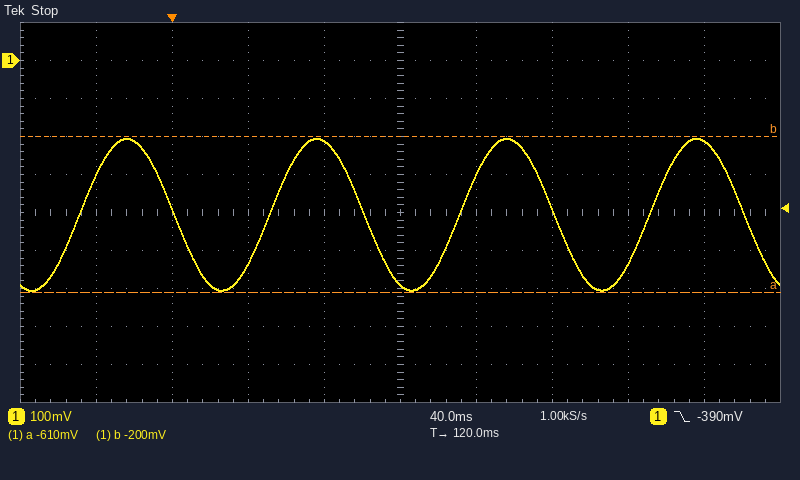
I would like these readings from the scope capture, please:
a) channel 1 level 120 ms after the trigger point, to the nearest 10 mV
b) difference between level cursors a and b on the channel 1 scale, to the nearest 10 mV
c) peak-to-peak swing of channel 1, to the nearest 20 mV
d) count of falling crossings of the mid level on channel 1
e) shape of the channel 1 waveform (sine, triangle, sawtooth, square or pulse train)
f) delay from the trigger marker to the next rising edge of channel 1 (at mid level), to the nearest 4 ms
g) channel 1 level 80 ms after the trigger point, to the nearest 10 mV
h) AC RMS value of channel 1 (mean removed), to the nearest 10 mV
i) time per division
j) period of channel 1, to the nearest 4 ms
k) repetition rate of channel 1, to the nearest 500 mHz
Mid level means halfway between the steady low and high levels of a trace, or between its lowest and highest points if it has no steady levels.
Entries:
-590 mV
410 mV
400 mV
4
sine
52 ms
-210 mV
140 mV
40 ms
100 ms
10.0 Hz
